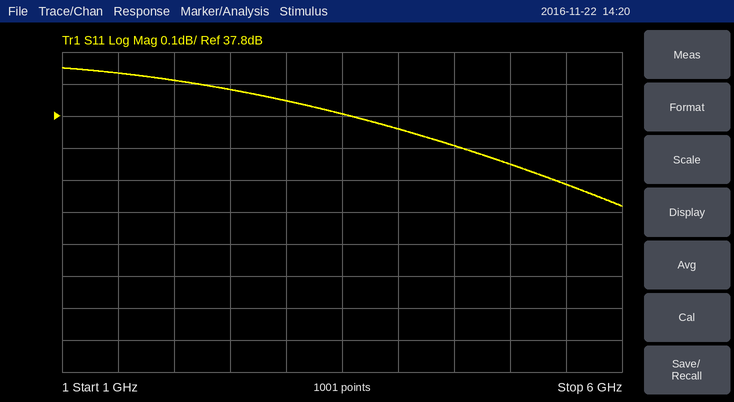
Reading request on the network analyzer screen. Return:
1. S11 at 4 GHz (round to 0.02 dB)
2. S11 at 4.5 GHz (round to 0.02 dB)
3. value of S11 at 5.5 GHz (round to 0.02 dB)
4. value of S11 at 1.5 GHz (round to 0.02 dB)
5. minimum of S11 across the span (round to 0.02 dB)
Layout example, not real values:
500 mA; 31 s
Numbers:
37.76 dB; 37.70 dB; 37.58 dB; 37.94 dB; 37.52 dB
